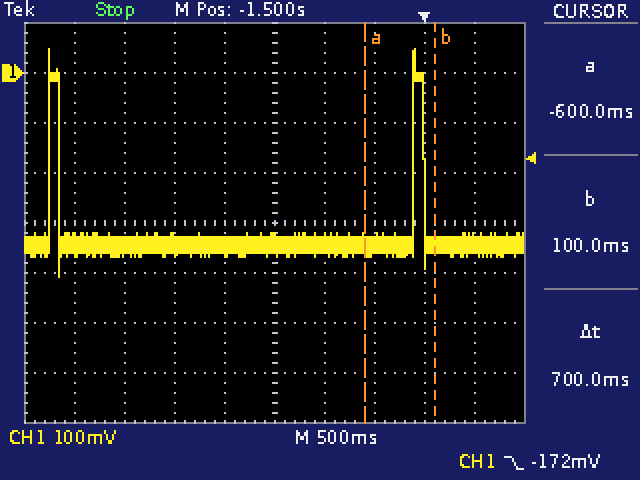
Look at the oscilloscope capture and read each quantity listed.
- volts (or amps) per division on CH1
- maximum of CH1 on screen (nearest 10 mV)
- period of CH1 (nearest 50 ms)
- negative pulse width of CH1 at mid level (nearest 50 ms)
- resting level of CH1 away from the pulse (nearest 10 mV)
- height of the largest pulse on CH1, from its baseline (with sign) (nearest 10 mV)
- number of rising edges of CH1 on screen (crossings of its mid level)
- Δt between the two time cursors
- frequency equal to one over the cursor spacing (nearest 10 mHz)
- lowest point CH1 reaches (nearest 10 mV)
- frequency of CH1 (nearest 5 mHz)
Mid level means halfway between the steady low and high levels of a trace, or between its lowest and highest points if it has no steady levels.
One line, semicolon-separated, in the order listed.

100 mV; 50 mV; 3.65 s; 3.55 s; -340 mV; +390 mV; 2; 700 ms; 1.43 Hz; -410 mV; 275 mHz
